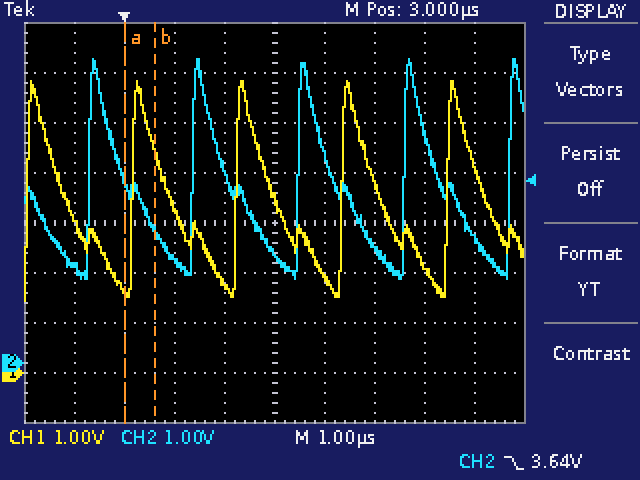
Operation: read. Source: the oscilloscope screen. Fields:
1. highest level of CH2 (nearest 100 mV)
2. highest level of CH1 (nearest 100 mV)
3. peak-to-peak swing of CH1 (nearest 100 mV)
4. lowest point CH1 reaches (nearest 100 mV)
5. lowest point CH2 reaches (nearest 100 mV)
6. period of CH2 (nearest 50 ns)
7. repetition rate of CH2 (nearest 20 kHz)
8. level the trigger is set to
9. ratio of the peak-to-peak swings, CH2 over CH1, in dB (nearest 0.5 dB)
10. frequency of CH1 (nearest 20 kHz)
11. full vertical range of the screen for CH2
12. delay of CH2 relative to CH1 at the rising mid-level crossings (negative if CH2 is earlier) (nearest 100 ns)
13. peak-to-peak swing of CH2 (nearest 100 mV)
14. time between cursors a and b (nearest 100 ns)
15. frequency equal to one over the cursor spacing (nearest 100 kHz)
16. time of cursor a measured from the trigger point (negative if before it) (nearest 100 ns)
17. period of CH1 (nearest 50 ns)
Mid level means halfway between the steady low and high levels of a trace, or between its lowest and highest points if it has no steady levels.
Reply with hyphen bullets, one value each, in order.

- 6.1 V
- 5.8 V
- 4.4 V
- 1.4 V
- 1.7 V
- 2.10 µs
- 480 kHz
- 3.64 V
- 0.0 dB
- 480 kHz
- 8 V
- -900 ns
- 4.4 V
- 600 ns
- 1.7 MHz
- 0.0 µs
- 2.10 µs
